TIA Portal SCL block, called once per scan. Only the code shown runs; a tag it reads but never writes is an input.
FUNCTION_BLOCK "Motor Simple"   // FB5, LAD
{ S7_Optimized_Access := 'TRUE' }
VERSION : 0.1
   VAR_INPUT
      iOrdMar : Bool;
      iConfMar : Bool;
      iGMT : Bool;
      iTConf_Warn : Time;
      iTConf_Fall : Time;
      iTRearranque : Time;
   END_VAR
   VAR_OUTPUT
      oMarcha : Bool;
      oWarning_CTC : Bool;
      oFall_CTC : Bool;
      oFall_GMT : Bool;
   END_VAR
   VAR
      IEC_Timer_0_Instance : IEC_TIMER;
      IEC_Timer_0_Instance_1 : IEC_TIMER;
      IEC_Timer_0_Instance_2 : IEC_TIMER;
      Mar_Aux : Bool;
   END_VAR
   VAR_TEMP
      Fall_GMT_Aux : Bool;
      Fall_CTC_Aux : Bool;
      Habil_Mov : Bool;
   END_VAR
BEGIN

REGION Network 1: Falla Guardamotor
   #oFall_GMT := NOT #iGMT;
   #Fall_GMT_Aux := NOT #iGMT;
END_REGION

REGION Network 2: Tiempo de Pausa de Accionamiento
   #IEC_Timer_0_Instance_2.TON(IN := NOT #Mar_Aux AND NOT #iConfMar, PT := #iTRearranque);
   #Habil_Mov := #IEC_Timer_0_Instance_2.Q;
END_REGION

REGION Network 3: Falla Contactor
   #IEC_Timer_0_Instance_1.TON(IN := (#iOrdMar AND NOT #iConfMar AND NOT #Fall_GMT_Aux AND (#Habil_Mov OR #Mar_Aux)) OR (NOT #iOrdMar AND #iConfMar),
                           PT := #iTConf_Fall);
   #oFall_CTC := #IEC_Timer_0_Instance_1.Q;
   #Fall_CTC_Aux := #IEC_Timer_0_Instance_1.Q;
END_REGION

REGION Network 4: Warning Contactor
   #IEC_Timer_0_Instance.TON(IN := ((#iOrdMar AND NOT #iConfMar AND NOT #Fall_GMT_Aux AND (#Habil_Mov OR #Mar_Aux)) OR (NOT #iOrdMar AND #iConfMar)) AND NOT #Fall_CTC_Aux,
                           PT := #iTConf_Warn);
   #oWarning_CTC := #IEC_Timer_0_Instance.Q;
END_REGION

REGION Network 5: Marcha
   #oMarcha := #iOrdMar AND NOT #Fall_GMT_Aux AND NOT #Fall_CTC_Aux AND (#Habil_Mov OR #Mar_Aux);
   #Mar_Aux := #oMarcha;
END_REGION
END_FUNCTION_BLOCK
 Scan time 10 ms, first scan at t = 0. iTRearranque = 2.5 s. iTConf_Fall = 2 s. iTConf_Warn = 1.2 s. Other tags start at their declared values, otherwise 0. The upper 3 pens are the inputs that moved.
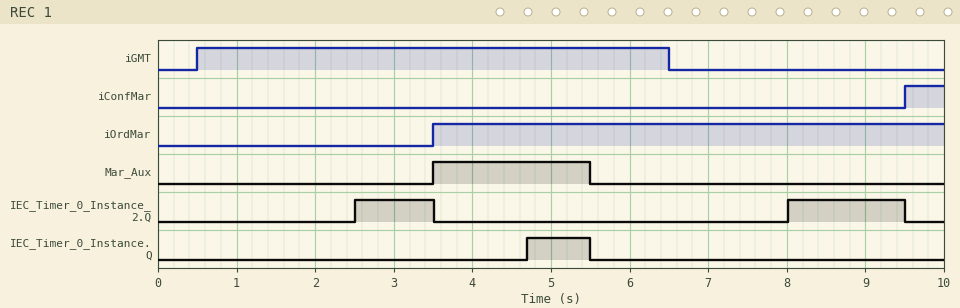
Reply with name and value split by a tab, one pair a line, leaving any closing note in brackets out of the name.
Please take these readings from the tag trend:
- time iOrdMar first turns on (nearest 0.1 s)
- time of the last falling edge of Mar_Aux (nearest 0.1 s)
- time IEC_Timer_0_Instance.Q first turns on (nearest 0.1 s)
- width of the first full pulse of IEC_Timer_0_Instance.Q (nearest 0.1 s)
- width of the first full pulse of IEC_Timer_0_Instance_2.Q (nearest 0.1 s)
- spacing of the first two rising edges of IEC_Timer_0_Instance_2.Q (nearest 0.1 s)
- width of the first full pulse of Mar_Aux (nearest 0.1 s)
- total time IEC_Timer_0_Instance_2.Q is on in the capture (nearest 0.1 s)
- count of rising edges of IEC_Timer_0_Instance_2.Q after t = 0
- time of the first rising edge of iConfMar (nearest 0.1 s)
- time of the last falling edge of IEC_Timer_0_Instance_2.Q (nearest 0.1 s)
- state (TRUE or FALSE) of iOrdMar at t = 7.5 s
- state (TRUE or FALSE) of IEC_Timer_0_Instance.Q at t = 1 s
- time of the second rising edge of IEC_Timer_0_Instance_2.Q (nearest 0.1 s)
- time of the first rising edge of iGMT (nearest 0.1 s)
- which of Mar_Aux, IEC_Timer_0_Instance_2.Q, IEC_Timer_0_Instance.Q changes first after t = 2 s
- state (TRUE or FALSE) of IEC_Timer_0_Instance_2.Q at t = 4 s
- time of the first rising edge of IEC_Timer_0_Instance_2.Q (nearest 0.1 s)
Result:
time iOrdMar first turns on	3.5 s
time of the last falling edge of Mar_Aux	5.5 s
time IEC_Timer_0_Instance.Q first turns on	4.7 s
width of the first full pulse of IEC_Timer_0_Instance.Q	0.8 s
width of the first full pulse of IEC_Timer_0_Instance_2.Q	1.0 s
spacing of the first two rising edges of IEC_Timer_0_Instance_2.Q	5.5 s
width of the first full pulse of Mar_Aux	2.0 s
total time IEC_Timer_0_Instance_2.Q is on in the capture	2.5 s
count of rising edges of IEC_Timer_0_Instance_2.Q after t = 0	2
time of the first rising edge of iConfMar	9.5 s
time of the last falling edge of IEC_Timer_0_Instance_2.Q	9.5 s
state (TRUE or FALSE) of iOrdMar at t = 7.5 s	TRUE
state (TRUE or FALSE) of IEC_Timer_0_Instance.Q at t = 1 s	FALSE
time of the second rising edge of IEC_Timer_0_Instance_2.Q	8.0 s
time of the first rising edge of iGMT	0.5 s
which of Mar_Aux, IEC_Timer_0_Instance_2.Q, IEC_Timer_0_Instance.Q changes first after t = 2 s	IEC_Timer_0_Instance_2.Q
state (TRUE or FALSE) of IEC_Timer_0_Instance_2.Q at t = 4 s	FALSE
time of the first rising edge of IEC_Timer_0_Instance_2.Q	2.5 s
